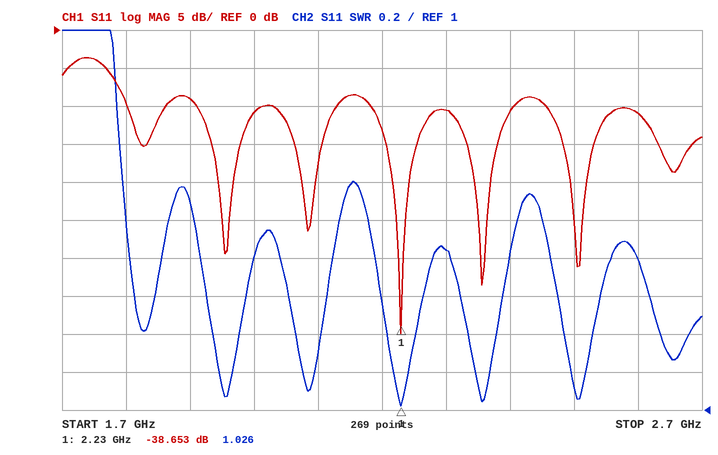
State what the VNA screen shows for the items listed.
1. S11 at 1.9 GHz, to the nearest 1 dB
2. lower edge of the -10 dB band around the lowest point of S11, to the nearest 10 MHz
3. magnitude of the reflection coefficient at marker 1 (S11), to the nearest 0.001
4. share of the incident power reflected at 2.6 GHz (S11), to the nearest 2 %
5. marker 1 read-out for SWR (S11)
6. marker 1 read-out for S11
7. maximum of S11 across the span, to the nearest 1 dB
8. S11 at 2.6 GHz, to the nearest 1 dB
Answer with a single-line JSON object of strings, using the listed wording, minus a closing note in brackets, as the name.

{"S11 at 1.9 GHz, to the nearest 1 dB": "-9 dB", "lower edge of the -10 dB band around the lowest point of S11, to the nearest 10 MHz": "2.18 GHz", "magnitude of the reflection coefficient at marker 1 (S11), to the nearest 0.001": "0.012", "share of the incident power reflected at 2.6 GHz (S11), to the nearest 2 %": "8 %", "marker 1 read-out for SWR": "1.026", "marker 1 read-out for S11": "-38.653 dB", "maximum of S11 across the span, to the nearest 1 dB": "-4 dB", "S11 at 2.6 GHz, to the nearest 1 dB": "-11 dB"}
